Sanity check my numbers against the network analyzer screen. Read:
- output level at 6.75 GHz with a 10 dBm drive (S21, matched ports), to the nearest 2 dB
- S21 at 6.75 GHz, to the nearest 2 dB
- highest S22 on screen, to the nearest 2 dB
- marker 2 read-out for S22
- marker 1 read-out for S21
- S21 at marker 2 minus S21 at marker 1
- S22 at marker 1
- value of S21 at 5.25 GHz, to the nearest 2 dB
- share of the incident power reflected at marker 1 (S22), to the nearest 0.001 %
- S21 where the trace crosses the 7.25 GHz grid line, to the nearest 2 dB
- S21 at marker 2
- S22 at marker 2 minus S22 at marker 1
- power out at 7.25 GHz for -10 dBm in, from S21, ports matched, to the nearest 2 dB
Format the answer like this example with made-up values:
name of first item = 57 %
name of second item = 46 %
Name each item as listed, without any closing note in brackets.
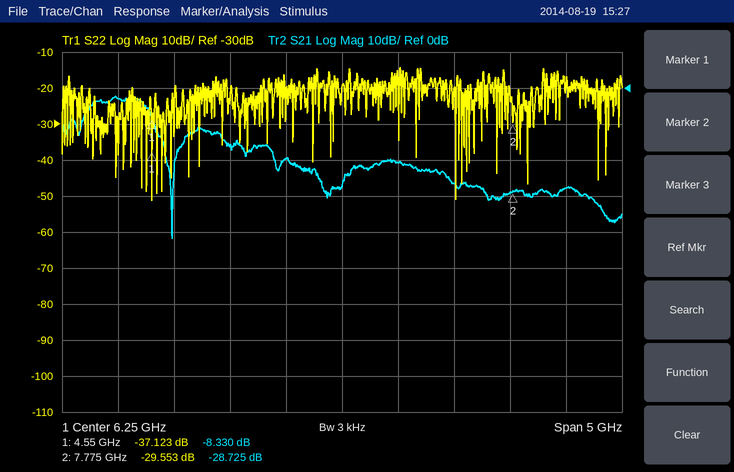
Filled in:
output level at 6.75 GHz with a 10 dBm drive (S21, matched ports), to the nearest 2 dB = -10 dBm
S21 at 6.75 GHz, to the nearest 2 dB = -20 dB
highest S22 on screen, to the nearest 2 dB = -14 dB
marker 2 read-out for S22 = -29.553 dB
marker 1 read-out for S21 = -8.330 dB
S21 at marker 2 minus S21 at marker 1 = -20.395 dB
S22 at marker 1 = -37.123 dB
value of S21 at 5.25 GHz, to the nearest 2 dB = -16 dB
share of the incident power reflected at marker 1 (S22), to the nearest 0.001 % = 0.019 %
S21 where the trace crosses the 7.25 GHz grid line, to the nearest 2 dB = -26 dB
S21 at marker 2 = -28.725 dB
S22 at marker 2 minus S22 at marker 1 = 7.570 dB
power out at 7.25 GHz for -10 dBm in, from S21, ports matched, to the nearest 2 dB = -36 dBm
